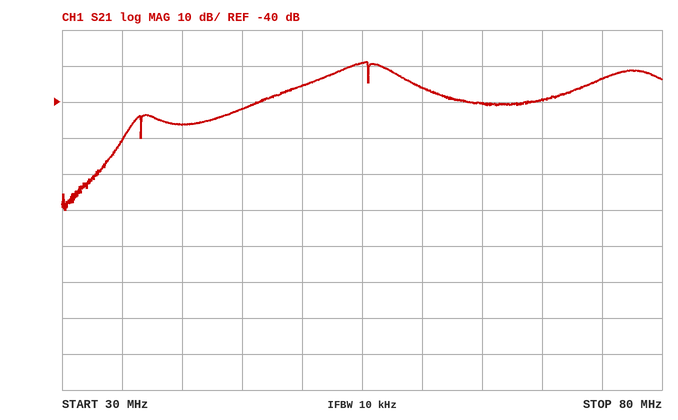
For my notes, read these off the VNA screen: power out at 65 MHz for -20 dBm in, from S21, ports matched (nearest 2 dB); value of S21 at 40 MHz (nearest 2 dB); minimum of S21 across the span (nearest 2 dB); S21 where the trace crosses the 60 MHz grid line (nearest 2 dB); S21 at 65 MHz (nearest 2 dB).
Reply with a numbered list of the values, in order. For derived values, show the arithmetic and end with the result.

1. -20 dBm + (-40 dB) = -60 dBm
2. -46 dB
3. -70 dB
4. -36 dB
5. -40 dB
